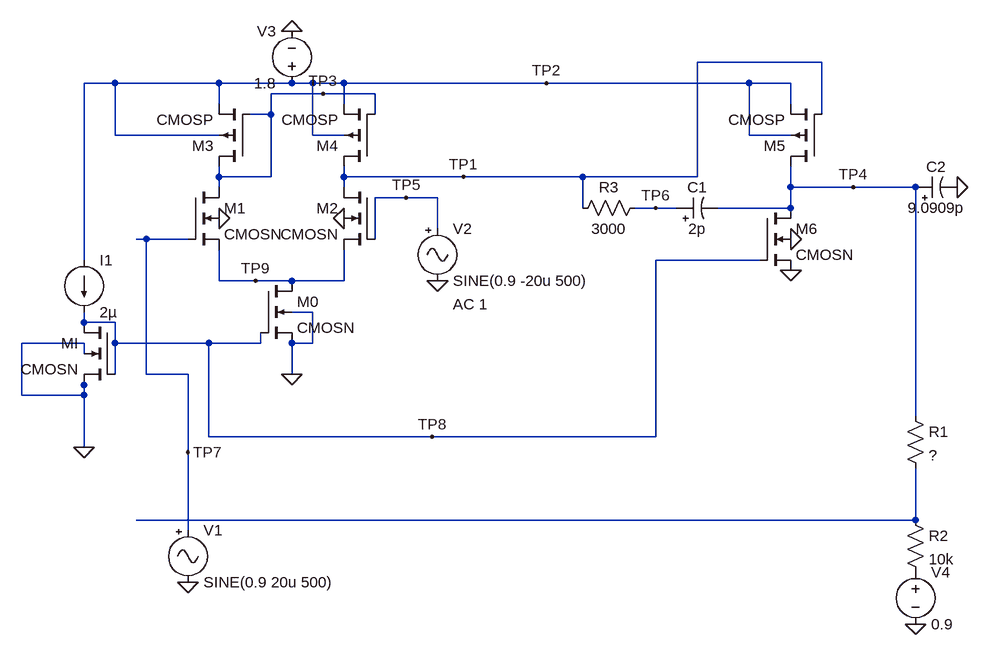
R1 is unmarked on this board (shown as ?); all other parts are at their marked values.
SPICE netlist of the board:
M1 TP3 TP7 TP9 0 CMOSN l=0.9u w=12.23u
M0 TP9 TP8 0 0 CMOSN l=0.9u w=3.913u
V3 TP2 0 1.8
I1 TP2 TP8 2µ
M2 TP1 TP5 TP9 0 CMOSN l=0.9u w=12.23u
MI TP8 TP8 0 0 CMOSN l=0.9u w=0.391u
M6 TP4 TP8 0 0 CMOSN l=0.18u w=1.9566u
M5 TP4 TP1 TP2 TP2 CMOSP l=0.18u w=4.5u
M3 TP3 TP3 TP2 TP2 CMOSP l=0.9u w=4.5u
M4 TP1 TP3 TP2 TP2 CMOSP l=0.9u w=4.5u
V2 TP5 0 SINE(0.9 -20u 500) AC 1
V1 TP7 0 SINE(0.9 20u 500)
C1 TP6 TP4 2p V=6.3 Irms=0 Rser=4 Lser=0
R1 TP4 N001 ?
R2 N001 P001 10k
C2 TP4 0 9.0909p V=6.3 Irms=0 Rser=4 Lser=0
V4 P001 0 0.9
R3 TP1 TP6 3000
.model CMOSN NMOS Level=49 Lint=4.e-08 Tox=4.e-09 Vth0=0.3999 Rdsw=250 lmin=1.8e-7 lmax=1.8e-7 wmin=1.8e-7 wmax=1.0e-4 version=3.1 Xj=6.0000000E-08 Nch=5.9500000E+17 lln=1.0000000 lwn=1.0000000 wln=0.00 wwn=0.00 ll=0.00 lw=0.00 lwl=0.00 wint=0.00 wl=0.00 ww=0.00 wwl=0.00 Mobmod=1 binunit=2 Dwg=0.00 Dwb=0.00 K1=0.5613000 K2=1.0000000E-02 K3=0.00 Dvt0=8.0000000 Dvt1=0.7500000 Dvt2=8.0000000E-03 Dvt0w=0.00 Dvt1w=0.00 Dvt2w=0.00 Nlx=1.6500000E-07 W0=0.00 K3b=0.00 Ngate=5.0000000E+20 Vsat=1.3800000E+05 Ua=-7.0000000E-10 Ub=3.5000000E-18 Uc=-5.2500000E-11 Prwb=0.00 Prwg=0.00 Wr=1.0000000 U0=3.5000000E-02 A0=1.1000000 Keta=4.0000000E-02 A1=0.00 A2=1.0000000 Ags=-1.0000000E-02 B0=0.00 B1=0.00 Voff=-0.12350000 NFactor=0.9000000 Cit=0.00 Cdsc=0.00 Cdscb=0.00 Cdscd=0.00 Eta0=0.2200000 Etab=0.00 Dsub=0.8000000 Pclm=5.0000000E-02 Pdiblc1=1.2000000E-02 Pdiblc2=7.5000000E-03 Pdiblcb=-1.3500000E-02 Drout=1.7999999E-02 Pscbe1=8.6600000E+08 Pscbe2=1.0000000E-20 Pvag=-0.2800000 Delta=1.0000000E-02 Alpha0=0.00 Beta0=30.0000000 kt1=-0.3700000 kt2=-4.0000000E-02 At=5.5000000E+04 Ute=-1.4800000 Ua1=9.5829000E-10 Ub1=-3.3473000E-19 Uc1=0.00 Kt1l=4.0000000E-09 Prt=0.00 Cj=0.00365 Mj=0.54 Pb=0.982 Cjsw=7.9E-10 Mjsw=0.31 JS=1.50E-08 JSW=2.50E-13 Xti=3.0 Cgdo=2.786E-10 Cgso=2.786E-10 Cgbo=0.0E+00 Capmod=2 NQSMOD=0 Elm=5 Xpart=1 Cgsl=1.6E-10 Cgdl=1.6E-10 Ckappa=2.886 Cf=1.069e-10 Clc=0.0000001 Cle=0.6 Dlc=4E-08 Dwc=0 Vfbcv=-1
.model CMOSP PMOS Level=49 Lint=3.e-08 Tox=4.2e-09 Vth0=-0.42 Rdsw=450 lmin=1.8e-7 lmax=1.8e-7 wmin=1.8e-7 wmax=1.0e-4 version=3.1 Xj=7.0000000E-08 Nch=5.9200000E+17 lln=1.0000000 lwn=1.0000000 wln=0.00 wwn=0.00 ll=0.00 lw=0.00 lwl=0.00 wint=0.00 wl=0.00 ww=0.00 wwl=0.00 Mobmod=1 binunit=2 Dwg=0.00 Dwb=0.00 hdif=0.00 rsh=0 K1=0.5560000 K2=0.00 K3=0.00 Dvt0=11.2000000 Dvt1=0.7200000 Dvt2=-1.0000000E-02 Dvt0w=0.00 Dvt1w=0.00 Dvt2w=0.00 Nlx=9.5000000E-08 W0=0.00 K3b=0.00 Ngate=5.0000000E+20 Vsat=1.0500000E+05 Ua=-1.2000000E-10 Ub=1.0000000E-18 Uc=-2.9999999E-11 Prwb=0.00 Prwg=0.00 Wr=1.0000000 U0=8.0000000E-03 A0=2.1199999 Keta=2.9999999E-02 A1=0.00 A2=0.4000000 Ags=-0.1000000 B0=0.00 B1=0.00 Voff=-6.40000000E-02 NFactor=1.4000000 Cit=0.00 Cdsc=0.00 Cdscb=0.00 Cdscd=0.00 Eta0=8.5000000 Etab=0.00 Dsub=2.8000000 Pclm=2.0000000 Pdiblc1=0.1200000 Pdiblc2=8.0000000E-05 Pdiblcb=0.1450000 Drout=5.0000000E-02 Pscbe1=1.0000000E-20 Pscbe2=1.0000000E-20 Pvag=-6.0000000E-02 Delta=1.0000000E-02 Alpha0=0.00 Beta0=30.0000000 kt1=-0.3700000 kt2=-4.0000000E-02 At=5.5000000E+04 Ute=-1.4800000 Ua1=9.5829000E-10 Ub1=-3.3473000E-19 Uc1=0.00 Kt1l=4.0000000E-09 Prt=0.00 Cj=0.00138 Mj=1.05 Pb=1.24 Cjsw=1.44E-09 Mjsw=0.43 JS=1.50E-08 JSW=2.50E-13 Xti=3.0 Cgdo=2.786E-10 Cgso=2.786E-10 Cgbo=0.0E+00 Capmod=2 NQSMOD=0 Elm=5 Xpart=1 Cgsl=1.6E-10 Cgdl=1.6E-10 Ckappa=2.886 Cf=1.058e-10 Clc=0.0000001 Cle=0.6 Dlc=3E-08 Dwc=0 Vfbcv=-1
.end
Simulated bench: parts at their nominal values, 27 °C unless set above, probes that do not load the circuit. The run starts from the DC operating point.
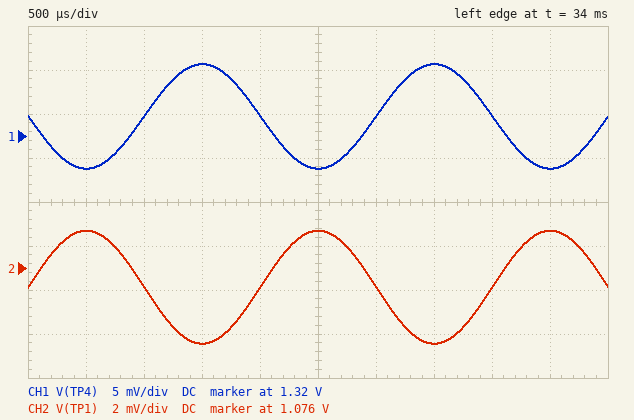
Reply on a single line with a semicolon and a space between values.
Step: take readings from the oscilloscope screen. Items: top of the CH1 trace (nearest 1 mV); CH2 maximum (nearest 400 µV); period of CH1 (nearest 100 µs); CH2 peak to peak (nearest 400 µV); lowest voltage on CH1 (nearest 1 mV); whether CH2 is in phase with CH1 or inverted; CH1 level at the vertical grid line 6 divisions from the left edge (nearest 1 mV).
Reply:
1.328 V; 1.0776 V; 2.0 ms; 5.2 mV; 1.316 V; inverted; 1.322 V
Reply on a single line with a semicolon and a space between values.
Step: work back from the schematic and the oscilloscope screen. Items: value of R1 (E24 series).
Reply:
3.3 kΩ
